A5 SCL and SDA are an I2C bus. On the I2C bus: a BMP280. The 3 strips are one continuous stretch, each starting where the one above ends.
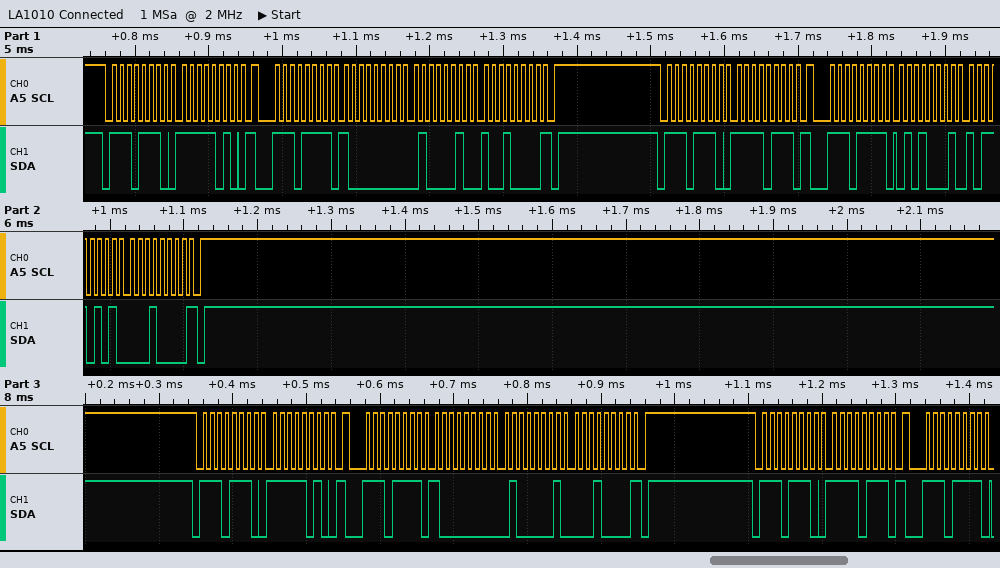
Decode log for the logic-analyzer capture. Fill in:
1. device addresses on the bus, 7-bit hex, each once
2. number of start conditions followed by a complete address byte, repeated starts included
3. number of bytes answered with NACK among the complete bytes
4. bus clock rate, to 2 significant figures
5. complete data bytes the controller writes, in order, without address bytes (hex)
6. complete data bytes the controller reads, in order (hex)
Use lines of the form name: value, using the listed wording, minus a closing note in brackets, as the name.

device addresses on the bus, 7-bit hex, each once: 0x77
number of start conditions followed by a complete address byte, repeated starts included: 8
number of bytes answered with NACK among the complete bytes: 3
bus clock rate, to 2 significant figures: 100 kHz
complete data bytes the controller writes, in order, without address bytes: FA F7 FA F7
complete data bytes the controller reads, in order: 80 42 90 51 B5 10 80 41 10
